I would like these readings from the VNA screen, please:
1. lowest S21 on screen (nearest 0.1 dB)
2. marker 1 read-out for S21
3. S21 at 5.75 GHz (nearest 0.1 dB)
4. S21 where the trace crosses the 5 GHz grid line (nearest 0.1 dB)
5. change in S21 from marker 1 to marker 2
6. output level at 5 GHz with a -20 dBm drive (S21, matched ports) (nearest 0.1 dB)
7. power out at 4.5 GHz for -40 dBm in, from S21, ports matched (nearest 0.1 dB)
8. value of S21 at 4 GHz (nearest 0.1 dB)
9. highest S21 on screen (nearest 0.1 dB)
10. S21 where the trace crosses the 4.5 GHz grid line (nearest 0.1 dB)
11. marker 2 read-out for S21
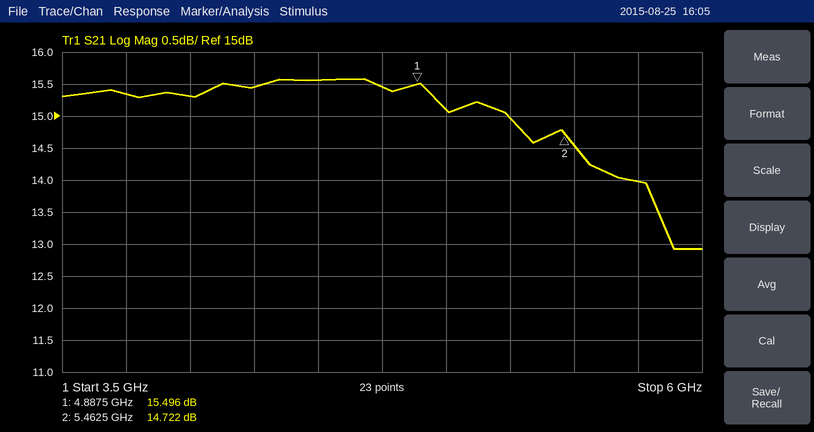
12.9 dB
15.496 dB
14.0 dB
15.1 dB
-0.774 dB
-4.9 dBm
-24.4 dBm
15.3 dB
15.6 dB
15.6 dB
14.722 dB
